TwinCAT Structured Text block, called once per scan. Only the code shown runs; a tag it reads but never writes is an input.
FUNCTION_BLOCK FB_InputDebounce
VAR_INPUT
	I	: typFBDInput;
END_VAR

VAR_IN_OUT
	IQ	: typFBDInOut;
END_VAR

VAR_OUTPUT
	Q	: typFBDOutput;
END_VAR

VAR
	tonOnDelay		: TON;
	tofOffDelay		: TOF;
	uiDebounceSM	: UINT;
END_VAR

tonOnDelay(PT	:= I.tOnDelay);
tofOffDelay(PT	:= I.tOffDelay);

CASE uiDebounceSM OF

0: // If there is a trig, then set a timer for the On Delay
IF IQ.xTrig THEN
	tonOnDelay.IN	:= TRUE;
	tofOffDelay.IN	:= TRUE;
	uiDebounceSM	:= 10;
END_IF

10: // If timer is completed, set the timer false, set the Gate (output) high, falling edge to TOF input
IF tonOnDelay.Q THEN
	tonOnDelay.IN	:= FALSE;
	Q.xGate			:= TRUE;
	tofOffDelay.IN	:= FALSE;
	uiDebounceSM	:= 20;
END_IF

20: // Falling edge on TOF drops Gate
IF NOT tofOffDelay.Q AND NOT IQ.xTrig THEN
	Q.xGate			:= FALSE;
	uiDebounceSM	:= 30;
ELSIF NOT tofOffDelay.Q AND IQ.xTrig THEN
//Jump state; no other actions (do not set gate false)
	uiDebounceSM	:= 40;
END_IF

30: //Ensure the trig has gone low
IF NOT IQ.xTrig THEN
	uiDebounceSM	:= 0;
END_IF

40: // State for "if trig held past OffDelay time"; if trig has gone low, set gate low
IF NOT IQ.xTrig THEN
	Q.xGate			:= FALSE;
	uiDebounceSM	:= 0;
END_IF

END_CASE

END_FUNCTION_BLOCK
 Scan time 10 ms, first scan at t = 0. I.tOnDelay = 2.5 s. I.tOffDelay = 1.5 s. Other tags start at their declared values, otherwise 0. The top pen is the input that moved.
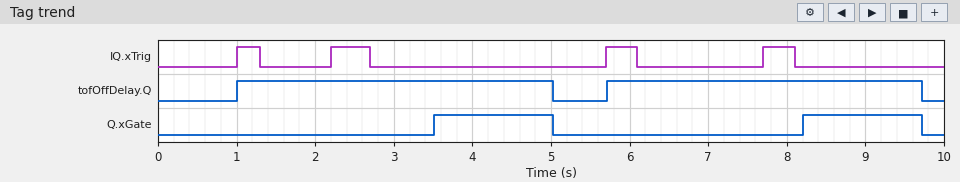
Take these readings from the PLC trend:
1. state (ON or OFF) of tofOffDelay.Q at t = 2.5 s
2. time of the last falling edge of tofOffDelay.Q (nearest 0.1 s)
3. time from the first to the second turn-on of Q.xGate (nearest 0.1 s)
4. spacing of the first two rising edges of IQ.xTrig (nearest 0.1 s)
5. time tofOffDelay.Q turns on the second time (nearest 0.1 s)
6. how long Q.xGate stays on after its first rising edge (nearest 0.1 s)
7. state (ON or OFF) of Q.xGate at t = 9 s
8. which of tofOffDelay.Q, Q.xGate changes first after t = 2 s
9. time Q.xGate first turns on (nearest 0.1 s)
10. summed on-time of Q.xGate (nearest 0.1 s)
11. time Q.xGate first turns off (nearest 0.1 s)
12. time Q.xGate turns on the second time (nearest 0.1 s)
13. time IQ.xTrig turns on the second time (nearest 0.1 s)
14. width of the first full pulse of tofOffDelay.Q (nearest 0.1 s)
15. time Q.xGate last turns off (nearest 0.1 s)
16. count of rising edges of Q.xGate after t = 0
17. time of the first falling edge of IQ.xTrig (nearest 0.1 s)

ON
9.7 s
4.7 s
1.2 s
5.7 s
1.5 s
ON
Q.xGate
3.5 s
3.0 s
5.0 s
8.2 s
2.2 s
4.0 s
9.7 s
2
1.3 s
